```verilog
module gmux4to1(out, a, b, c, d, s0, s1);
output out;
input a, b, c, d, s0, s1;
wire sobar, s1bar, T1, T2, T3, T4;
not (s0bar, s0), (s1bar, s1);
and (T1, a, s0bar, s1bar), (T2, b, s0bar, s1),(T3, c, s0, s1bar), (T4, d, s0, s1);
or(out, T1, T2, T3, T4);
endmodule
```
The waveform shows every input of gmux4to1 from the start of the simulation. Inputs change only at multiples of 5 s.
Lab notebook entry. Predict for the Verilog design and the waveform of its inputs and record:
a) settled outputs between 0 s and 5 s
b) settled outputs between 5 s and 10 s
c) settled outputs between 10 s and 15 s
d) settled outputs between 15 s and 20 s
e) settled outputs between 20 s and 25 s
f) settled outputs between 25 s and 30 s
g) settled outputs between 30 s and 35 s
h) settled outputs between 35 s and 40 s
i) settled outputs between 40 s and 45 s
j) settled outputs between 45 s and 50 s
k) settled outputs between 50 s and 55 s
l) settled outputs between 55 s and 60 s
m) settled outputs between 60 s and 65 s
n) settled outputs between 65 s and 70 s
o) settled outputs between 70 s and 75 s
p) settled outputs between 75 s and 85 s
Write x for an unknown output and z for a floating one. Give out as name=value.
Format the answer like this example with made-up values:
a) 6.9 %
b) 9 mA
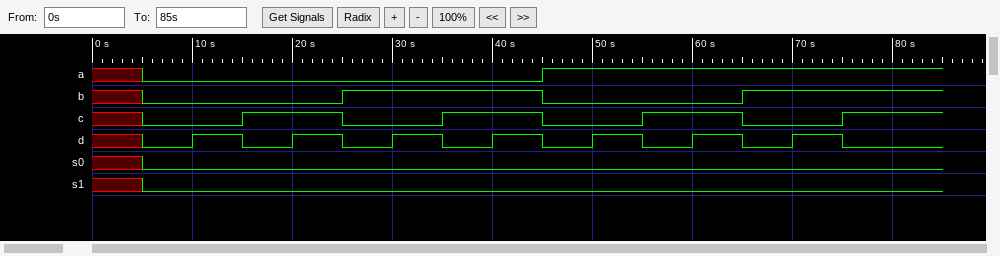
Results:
a) out=x
b) out=0
c) out=0
d) out=0
e) out=0
f) out=0
g) out=0
h) out=0
i) out=0
j) out=1
k) out=1
l) out=1
m) out=1
n) out=1
o) out=1
p) out=1
